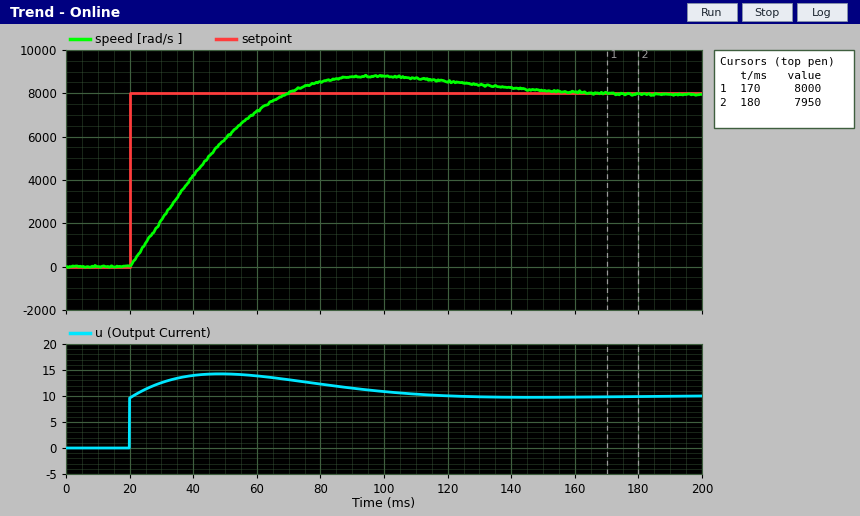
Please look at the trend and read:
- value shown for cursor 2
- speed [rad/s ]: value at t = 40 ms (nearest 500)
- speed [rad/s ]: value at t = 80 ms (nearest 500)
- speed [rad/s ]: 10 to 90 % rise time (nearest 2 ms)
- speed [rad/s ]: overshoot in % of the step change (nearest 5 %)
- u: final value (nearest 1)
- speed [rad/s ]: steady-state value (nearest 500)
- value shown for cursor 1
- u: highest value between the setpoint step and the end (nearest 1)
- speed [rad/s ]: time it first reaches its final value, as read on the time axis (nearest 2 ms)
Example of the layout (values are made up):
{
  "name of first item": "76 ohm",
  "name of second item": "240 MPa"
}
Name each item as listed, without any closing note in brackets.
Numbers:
{
  "value shown for cursor 2": "7950",
  "speed [rad/s ]: value at t = 40 ms": "4000",
  "speed [rad/s ]: value at t = 80 ms": "8500",
  "speed [rad/s ]: 10 to 90 % rise time": "36 ms",
  "speed [rad/s ]: overshoot in % of the step change": "10 %",
  "u: final value": "10",
  "speed [rad/s ]: steady-state value": "8000",
  "value shown for cursor 1": "8000",
  "u: highest value between the setpoint step and the end": "14",
  "speed [rad/s ]: time it first reaches its final value, as read on the time axis": "70 ms"
}
